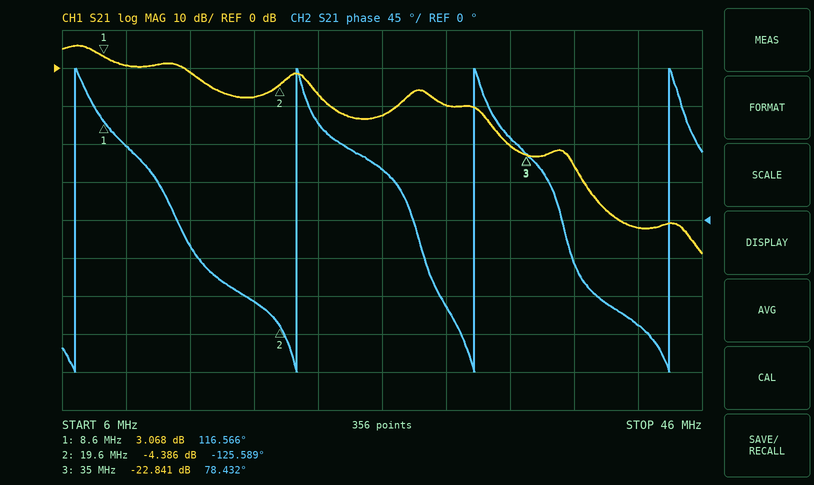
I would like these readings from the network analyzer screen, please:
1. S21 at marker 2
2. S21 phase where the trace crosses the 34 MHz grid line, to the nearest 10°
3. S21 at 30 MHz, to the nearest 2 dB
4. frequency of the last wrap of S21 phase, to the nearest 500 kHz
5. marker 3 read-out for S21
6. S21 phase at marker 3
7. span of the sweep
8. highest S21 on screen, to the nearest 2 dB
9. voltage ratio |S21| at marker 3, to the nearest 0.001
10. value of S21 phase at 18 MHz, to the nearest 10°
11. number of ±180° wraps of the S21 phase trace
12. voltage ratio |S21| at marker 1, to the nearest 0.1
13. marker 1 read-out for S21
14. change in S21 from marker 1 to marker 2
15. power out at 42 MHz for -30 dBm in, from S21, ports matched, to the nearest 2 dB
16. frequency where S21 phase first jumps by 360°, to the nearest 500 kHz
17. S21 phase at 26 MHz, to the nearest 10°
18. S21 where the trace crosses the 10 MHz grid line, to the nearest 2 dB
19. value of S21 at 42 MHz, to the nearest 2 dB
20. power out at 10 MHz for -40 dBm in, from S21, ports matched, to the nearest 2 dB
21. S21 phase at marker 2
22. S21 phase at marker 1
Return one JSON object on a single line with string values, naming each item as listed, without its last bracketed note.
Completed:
{"S21 at marker 2": "-4.386 dB", "S21 phase where the trace crosses the 34 MHz grid line, to the nearest 10°": "100°", "S21 at 30 MHz, to the nearest 2 dB": "-10 dB", "frequency of the last wrap of S21 phase, to the nearest 500 kHz": "44.0 MHz", "marker 3 read-out for S21": "-22.841 dB", "S21 phase at marker 3": "78.432°", "span of the sweep": "40 MHz", "highest S21 on screen, to the nearest 2 dB": "6 dB", "voltage ratio |S21| at marker 3, to the nearest 0.001": "0.072", "value of S21 phase at 18 MHz, to the nearest 10°": "-100°", "number of ±180° wraps of the S21 phase trace": "4", "voltage ratio |S21| at marker 1, to the nearest 0.1": "1.4", "marker 1 read-out for S21": "3.068 dB", "change in S21 from marker 1 to marker 2": "-7.454 dB", "power out at 42 MHz for -30 dBm in, from S21, ports matched, to the nearest 2 dB": "-72 dBm", "frequency where S21 phase first jumps by 360°, to the nearest 500 kHz": "7.0 MHz", "S21 phase at 26 MHz, to the nearest 10°": "60°", "S21 where the trace crosses the 10 MHz grid line, to the nearest 2 dB": "0 dB", "value of S21 at 42 MHz, to the nearest 2 dB": "-42 dB", "power out at 10 MHz for -40 dBm in, from S21, ports matched, to the nearest 2 dB": "-40 dBm", "S21 phase at marker 2": "-125.589°", "S21 phase at marker 1": "116.566°"}
